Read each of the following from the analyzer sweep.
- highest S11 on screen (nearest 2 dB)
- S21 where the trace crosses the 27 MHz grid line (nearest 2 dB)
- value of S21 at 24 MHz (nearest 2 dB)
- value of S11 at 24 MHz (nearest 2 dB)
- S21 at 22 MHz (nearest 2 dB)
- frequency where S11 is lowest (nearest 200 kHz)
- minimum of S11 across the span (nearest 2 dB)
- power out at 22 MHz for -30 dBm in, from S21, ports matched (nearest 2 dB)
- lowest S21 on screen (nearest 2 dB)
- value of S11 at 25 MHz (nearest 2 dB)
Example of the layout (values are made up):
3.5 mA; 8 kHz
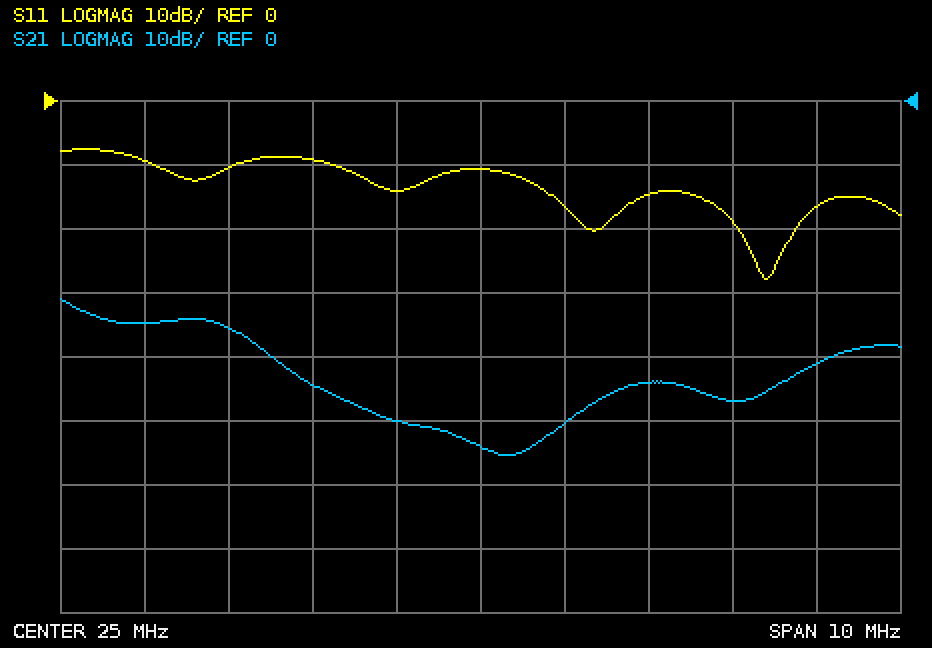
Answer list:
-8 dB; -44 dB; -50 dB; -14 dB; -36 dB; 28.4 MHz; -28 dB; -66 dBm; -56 dB; -10 dB
